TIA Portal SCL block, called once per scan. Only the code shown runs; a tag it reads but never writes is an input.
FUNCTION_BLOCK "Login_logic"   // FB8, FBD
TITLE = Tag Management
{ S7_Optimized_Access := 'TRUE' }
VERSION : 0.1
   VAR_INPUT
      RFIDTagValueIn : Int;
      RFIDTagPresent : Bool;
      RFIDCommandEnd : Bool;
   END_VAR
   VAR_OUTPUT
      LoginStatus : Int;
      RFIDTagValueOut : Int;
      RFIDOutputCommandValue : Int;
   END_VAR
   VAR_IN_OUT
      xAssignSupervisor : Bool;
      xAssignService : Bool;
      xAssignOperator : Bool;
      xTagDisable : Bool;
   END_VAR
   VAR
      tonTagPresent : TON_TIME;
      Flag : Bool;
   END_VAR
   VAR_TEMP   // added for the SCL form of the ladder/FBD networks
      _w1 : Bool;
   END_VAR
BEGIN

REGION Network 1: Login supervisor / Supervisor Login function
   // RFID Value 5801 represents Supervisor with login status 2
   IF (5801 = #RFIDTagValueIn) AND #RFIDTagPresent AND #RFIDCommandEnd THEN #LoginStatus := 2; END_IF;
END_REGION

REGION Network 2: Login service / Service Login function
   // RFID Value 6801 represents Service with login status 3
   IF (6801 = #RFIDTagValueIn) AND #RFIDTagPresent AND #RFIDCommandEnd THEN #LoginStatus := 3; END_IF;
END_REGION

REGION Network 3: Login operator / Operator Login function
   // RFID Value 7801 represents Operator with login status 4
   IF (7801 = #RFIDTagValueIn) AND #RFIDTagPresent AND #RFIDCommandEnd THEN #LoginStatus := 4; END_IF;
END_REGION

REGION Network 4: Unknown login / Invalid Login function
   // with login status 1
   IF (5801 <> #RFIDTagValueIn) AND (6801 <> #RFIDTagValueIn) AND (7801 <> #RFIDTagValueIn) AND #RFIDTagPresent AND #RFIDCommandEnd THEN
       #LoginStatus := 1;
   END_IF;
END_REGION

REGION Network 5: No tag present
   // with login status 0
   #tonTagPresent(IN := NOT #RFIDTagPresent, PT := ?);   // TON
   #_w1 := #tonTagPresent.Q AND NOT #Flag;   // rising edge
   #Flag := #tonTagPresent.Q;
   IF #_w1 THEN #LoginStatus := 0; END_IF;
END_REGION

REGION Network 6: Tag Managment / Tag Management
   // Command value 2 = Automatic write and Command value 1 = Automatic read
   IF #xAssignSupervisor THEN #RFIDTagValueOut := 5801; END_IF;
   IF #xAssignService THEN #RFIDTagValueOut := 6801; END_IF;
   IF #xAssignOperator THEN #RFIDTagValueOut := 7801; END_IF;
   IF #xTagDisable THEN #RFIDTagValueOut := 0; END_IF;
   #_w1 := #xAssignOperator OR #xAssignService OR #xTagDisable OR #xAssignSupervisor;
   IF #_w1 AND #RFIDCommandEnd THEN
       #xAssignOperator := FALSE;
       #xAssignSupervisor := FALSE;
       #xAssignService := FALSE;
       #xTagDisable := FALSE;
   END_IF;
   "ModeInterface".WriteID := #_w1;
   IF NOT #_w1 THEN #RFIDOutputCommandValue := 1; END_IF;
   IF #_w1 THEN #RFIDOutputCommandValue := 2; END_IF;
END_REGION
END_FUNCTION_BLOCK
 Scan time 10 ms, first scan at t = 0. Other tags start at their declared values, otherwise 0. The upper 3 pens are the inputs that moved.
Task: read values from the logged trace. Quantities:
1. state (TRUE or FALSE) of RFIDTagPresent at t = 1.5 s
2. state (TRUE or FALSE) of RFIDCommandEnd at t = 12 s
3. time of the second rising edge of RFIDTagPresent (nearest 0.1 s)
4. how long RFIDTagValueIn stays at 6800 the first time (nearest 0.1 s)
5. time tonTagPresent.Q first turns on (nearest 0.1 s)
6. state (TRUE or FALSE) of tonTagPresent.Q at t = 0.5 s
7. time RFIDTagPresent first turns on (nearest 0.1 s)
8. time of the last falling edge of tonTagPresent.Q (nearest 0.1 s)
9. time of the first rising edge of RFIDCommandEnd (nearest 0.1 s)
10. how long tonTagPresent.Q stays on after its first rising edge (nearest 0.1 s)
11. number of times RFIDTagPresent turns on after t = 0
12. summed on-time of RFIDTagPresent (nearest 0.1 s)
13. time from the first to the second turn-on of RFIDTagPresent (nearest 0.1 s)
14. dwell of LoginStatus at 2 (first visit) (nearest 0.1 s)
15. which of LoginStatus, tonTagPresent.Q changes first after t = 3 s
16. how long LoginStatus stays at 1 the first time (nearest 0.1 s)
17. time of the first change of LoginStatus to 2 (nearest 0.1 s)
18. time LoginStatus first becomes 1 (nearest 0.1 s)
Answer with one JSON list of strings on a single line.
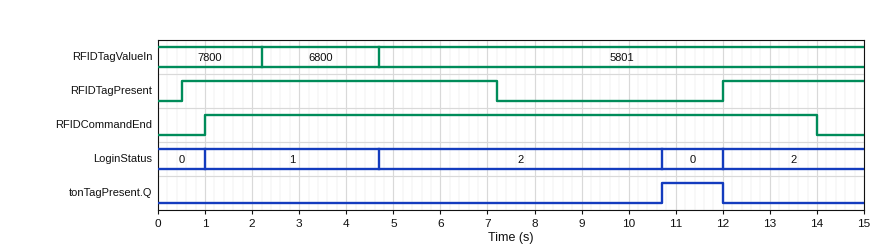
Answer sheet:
["TRUE", "TRUE", "12.0 s", "2.5 s", "10.7 s", "FALSE", "0.5 s", "12.0 s", "1.0 s", "1.3 s", "2", "9.7 s", "11.5 s", "6.0 s", "LoginStatus", "3.7 s", "4.7 s", "1.0 s"]
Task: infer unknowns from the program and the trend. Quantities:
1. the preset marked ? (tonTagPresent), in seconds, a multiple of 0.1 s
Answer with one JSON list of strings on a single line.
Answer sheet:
["3.5 s"]
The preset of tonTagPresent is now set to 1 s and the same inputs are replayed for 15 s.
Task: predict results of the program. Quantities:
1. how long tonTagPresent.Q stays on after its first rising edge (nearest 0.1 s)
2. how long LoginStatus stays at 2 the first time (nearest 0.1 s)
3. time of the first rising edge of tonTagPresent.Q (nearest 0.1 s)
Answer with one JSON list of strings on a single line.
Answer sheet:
["3.8 s", "3.5 s", "8.2 s"]
